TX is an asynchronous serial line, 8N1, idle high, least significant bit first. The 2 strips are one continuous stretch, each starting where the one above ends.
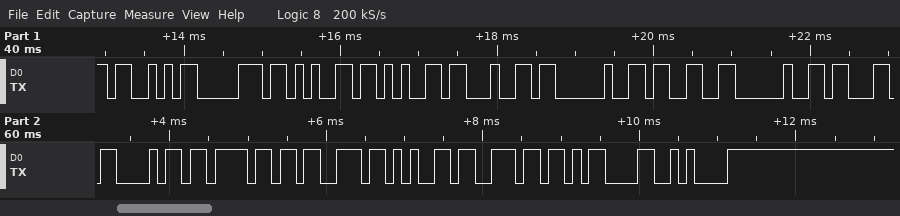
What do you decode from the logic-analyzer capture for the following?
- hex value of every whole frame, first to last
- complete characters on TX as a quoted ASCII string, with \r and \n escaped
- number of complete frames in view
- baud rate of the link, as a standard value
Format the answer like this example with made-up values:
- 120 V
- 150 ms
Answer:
- 53 70 65 65 64 20 33 20 63 68 6F 73 65 6E 0D 0A
- "Speed 3 chosen\r\n"
- 16
- 9600 baud
